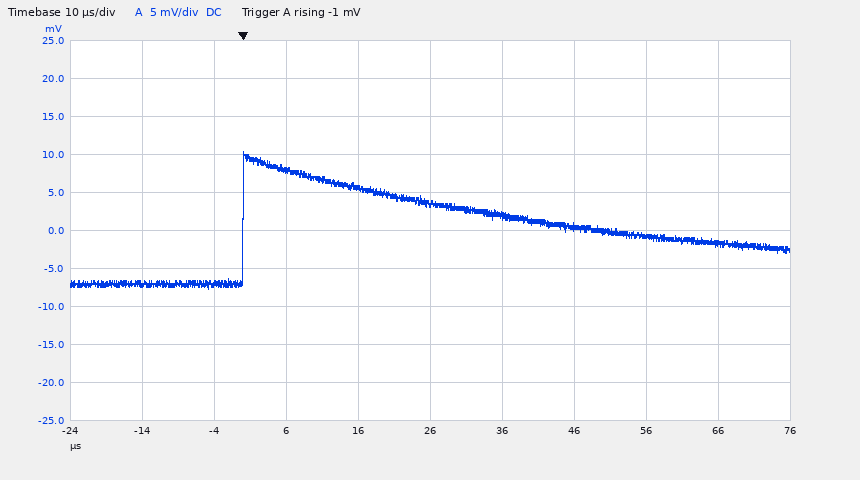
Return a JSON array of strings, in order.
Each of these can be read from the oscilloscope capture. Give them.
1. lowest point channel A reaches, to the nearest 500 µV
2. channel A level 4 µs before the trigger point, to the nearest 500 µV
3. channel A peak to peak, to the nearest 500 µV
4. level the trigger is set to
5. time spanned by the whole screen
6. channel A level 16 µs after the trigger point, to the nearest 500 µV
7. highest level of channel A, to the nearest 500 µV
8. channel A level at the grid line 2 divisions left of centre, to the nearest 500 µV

["-7.5 mV", "-7.0 mV", "18.0 mV", "-1 mV", "100 µs", "5.5 mV", "10.5 mV", "8.0 mV"]
